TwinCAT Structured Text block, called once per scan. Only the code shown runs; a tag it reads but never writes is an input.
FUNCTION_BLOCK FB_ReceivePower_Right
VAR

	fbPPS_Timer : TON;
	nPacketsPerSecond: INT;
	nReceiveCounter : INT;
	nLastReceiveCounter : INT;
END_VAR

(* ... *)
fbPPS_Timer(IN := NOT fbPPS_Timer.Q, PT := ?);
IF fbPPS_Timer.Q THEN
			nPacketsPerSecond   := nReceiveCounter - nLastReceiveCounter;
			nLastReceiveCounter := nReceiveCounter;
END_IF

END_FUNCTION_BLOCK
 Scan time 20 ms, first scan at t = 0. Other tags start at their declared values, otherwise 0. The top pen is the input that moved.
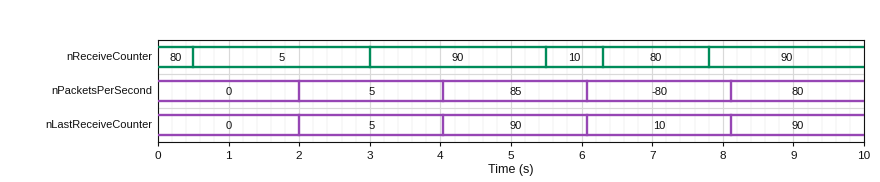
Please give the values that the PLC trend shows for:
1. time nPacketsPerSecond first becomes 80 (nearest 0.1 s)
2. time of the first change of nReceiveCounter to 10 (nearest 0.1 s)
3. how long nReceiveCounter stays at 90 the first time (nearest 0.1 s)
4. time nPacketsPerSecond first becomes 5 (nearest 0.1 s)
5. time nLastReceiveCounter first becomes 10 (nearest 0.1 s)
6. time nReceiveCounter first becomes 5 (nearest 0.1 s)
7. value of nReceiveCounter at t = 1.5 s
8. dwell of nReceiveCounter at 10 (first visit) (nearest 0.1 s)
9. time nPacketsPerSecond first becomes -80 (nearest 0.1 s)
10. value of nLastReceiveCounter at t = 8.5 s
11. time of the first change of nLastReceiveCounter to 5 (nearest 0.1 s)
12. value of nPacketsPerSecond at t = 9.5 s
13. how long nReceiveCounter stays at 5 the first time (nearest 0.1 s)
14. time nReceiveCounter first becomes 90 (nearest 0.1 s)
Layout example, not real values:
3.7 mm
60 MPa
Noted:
8.1 s
5.5 s
2.5 s
2.0 s
6.1 s
0.5 s
5
0.8 s
6.1 s
90
2.0 s
80
2.5 s
3.0 s
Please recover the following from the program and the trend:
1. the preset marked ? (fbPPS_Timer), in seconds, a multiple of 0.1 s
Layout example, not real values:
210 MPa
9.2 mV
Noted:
2.0 s
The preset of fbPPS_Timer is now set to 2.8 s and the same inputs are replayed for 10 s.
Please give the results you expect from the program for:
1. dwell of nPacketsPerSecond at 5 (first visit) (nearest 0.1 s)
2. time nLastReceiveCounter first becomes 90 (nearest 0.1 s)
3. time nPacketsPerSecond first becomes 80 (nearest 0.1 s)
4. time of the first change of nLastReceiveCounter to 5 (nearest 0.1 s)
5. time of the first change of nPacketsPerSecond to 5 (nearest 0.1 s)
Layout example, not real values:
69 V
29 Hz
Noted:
5.7 s
8.5 s
8.5 s
2.8 s
2.8 s
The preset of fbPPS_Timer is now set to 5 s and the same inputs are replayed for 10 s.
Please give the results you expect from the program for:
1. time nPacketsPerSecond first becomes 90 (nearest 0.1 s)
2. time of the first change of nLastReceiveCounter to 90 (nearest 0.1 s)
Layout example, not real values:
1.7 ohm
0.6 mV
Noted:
5.0 s
5.0 s
